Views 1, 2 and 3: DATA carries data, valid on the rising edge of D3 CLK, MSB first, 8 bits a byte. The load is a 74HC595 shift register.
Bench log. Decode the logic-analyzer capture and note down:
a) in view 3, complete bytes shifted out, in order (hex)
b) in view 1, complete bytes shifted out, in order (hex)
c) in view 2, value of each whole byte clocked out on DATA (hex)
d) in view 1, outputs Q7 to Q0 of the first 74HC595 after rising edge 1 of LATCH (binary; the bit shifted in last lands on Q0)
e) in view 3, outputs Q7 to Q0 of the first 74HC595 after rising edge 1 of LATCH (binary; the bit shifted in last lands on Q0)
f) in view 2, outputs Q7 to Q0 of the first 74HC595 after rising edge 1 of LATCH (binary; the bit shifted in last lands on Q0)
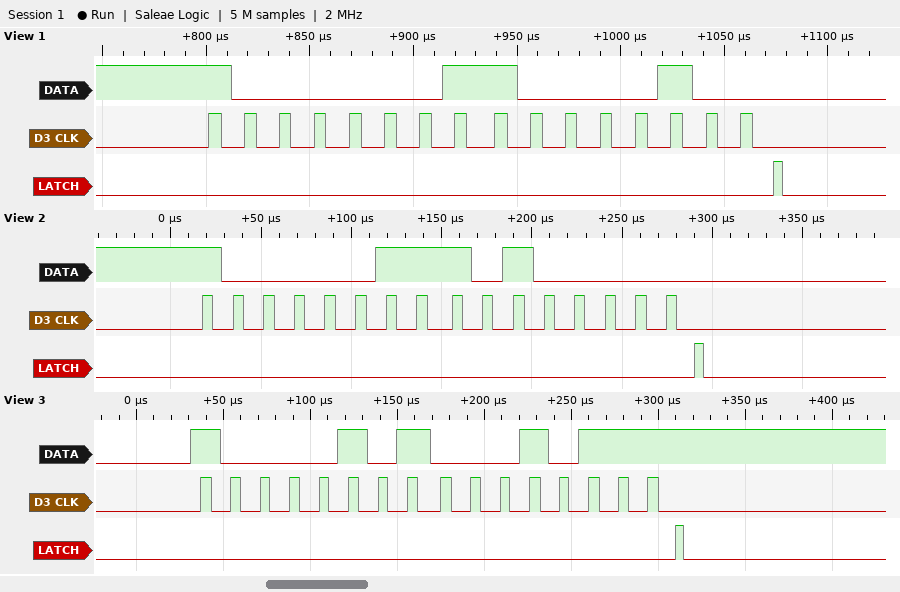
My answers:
85 17
81 84
83 A0
10000100
00010111
10100000
